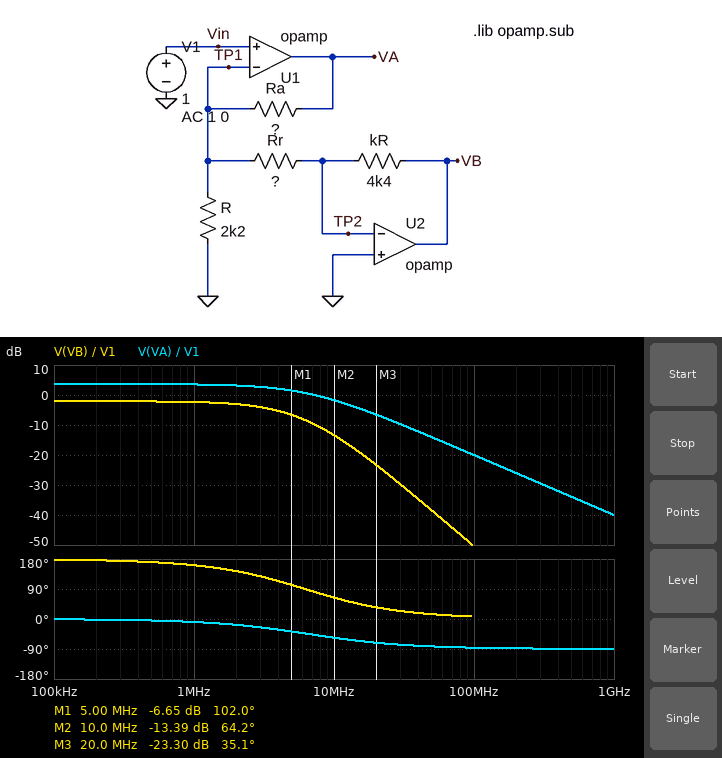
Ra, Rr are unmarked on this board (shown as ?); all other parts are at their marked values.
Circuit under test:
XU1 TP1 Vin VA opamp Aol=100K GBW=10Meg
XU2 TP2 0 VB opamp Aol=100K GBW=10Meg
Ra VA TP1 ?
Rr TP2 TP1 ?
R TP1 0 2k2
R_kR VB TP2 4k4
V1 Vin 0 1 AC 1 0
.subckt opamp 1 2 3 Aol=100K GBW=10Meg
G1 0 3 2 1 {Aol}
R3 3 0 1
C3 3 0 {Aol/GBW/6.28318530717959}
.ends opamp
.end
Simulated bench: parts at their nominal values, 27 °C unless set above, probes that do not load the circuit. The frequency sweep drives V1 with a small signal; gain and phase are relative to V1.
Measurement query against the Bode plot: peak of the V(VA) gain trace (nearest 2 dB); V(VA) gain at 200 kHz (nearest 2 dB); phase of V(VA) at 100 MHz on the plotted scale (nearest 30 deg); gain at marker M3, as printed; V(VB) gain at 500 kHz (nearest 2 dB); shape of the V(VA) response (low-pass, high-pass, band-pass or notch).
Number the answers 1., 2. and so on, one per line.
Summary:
1. 4 dB
2. 4 dB
3. -90 deg
4. -23.30 dB
5. -2 dB
6. low-pass
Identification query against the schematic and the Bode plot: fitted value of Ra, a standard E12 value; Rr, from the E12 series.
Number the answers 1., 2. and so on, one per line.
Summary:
1. 820 Ω
2. 5.6 kΩ
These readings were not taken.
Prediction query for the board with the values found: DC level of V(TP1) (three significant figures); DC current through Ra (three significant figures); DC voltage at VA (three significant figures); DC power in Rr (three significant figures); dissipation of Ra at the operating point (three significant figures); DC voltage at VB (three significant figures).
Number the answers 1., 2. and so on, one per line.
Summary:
1. 1.00 V
2. 633 µA
3. 1.52 V
4. 179 µW
5. 329 µW
6. -786 mV
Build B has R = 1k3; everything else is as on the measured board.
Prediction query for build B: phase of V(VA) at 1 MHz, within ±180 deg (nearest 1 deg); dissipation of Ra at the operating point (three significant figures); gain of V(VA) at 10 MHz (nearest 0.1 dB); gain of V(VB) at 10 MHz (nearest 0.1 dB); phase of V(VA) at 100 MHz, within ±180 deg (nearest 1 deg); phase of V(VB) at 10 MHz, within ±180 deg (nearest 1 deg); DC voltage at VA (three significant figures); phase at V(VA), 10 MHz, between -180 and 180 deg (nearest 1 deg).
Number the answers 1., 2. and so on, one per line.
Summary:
1. -10 deg
2. 737 µW
3. -1.3 dB
4. -14.4 dB
5. -87 deg
6. 60 deg
7. 1.78 V
8. -60 deg
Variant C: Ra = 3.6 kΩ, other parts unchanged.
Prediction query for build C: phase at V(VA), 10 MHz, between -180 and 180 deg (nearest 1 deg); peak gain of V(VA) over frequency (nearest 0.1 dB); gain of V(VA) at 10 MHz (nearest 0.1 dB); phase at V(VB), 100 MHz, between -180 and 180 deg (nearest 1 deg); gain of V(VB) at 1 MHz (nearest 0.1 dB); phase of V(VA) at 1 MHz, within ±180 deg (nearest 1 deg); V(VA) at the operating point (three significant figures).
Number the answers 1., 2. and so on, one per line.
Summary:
1. -72 deg
2. 10.3 dB
3. -0.5 dB
4. 5 deg
5. -2.7 dB
6. -19 deg
7. 3.28 V
